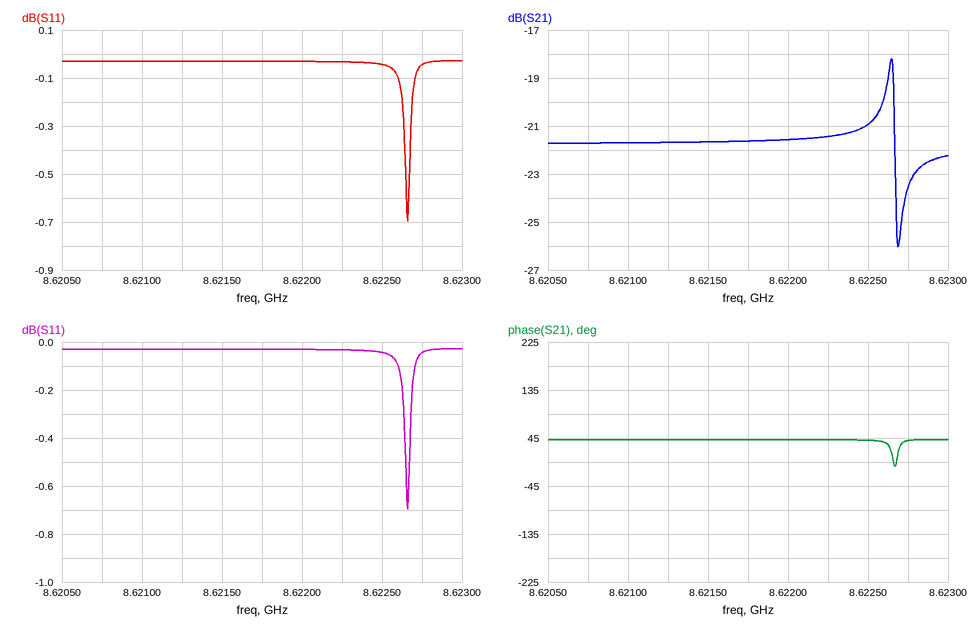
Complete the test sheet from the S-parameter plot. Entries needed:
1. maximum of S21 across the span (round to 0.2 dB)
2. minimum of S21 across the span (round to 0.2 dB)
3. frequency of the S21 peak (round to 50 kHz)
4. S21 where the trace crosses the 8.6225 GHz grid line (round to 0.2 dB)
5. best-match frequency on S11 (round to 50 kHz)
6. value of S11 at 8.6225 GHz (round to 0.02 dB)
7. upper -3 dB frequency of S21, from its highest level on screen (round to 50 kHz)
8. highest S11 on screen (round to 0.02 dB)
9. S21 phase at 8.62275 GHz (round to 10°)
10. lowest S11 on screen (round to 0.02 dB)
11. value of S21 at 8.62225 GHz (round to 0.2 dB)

-18.2 dB
-26.0 dB
8.62265 GHz
-21.0 dB
8.62265 GHz
-0.04 dB
8.62265 GHz
-0.02 dB
40°
-0.70 dB
-21.4 dB
